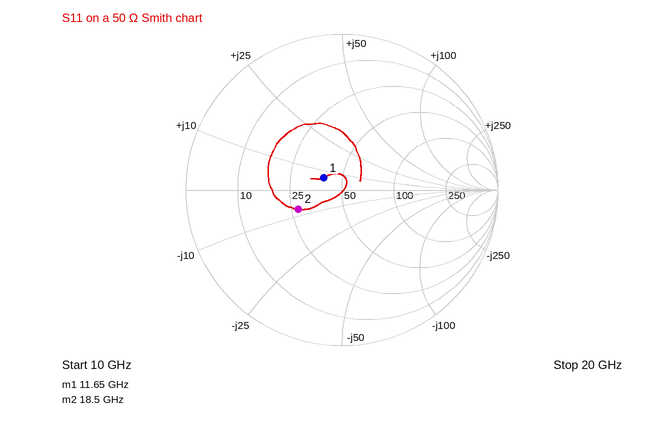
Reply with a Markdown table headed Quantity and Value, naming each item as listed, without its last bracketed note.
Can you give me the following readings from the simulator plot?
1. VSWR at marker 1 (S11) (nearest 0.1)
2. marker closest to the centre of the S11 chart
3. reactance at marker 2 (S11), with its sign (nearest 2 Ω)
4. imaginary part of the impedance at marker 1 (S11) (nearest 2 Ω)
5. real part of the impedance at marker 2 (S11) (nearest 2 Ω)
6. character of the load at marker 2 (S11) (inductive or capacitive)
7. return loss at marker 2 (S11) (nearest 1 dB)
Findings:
| Quantity | Value |
|---|---|
| VSWR at marker 1 (S11) | 1.3 |
| marker closest to the centre of the S11 chart | marker 1 |
| reactance at marker 2 (S11), with its sign | -8 Ω |
| imaginary part of the impedance at marker 1 (S11) | +6 Ω |
| real part of the impedance at marker 2 (S11) | 28 Ω |
| character of the load at marker 2 (S11) | capacitive |
| return loss at marker 2 (S11) | 10 dB |
